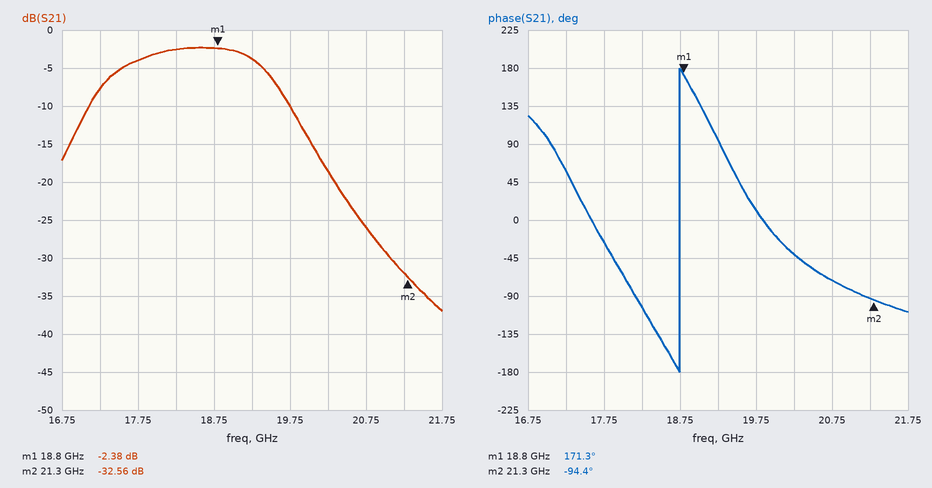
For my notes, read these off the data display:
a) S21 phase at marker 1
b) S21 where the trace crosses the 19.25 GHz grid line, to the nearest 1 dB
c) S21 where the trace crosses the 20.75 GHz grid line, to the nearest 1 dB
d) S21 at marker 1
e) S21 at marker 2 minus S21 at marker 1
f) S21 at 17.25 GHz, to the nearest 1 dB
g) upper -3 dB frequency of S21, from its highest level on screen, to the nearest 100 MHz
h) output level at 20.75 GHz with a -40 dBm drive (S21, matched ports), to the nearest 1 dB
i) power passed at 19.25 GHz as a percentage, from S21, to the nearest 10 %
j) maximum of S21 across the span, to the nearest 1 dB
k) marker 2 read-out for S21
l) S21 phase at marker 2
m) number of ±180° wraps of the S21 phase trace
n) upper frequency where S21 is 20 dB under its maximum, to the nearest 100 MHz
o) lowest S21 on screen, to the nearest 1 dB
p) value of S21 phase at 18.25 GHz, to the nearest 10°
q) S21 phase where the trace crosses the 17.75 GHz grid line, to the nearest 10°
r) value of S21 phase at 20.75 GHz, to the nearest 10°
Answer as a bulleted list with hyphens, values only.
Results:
- 171.3°
- -4 dB
- -26 dB
- -2.38 dB
- -30.18 dB
- -8 dB
- 19.4 GHz
- -66 dBm
- 40 %
- -2 dB
- -32.56 dB
- -94.4°
- 1
- 20.5 GHz
- -37 dB
- -100°
- -30°
- -70°
